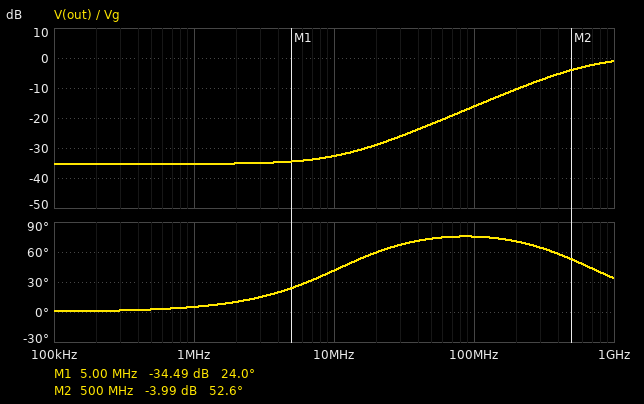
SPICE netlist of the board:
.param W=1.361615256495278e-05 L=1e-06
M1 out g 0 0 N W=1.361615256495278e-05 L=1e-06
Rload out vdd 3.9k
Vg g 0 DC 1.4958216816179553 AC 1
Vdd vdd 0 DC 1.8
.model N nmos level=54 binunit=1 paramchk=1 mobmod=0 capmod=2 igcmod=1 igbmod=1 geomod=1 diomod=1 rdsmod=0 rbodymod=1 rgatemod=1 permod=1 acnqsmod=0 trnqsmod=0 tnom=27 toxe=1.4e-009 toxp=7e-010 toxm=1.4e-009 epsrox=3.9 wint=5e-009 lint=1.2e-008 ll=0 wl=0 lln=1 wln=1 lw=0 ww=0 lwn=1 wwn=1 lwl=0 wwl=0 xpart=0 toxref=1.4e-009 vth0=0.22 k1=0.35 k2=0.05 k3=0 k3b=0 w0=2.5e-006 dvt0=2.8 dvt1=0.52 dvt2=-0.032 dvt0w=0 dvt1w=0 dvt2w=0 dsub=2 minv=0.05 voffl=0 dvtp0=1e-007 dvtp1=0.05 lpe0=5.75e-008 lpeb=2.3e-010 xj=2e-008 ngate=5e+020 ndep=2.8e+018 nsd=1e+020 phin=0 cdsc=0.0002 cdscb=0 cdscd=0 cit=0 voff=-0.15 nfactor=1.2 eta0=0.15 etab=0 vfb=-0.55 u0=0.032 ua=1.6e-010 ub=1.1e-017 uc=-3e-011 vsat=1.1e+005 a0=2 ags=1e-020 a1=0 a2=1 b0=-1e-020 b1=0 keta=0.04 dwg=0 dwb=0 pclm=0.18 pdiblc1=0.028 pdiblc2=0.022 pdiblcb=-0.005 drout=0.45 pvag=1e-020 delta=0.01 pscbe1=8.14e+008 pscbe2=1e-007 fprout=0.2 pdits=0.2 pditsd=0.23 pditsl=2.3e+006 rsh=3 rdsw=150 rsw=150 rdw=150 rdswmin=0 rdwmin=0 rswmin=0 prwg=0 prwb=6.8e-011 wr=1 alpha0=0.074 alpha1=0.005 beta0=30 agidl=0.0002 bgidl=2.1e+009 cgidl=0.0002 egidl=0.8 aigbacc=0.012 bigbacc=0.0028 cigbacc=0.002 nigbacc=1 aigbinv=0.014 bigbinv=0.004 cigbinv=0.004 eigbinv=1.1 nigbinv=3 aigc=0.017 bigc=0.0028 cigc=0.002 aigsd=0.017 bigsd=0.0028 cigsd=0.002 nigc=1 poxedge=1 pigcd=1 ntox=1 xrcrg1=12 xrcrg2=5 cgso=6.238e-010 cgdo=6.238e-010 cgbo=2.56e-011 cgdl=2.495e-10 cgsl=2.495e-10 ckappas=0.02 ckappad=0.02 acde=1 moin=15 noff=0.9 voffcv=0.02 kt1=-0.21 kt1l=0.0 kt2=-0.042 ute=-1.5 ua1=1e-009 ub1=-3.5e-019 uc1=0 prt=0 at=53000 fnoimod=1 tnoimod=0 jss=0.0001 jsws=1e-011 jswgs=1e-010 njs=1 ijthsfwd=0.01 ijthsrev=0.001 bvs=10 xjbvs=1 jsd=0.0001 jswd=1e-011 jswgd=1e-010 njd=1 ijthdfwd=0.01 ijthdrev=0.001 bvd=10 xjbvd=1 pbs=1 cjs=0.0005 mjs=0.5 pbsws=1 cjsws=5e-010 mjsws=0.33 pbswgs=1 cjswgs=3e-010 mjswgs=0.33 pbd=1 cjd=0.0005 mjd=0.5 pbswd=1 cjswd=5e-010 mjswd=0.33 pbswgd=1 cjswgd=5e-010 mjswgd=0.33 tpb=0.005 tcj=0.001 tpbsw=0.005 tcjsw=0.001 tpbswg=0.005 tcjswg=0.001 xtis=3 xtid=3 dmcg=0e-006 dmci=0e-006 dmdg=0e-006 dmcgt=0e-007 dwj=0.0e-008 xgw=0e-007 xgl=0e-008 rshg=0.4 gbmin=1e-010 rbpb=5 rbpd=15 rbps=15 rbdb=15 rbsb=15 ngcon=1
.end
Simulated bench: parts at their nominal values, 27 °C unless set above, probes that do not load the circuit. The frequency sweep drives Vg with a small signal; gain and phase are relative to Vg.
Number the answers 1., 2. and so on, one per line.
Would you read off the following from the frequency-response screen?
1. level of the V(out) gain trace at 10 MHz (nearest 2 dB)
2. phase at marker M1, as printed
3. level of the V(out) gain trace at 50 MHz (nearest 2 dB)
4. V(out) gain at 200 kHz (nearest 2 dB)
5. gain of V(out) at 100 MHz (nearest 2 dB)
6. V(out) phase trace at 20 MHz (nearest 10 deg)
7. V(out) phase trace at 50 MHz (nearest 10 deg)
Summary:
1. -32 dB
2. 24.0 deg
3. -22 dB
4. -36 dB
5. -16 dB
6. 60 deg
7. 70 deg
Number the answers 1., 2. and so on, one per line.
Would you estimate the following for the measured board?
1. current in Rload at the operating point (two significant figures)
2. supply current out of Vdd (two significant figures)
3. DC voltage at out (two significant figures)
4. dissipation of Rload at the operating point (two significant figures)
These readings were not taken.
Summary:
1. 370 µA
2. 370 µA
3. 360 mV
4. 530 µW
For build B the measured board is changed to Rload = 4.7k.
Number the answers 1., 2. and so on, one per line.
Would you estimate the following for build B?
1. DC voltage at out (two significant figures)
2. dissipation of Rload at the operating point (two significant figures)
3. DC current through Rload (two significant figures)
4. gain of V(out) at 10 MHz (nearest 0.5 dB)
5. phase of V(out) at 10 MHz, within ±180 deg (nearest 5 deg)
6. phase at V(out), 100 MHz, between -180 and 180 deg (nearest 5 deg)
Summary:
1. 300 mV
2. 480 µW
3. 320 µA
4. -29.5 dB
5. 25 deg
6. 70 deg
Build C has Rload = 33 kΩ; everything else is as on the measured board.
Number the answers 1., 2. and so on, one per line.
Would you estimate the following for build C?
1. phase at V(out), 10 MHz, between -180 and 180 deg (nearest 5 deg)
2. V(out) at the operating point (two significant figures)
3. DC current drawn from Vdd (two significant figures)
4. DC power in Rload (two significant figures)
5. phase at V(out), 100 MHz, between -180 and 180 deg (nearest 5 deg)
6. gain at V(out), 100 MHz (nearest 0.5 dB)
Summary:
1. 30 deg
2. 46 mV
3. 53 µA
4. 93 µW
5. 70 deg
6. -17.0 dB
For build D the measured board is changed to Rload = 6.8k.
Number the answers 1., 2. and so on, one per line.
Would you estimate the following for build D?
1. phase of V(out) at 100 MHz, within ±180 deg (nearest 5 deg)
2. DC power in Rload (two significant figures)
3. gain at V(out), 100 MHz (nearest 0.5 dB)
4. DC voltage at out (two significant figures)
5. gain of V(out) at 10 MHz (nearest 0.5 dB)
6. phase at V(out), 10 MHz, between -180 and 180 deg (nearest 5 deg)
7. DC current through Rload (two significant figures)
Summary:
1. 65 deg
2. 370 µW
3. -16.5 dB
4. 210 mV
5. -28.0 dB
6. 20 deg
7. 230 µA
